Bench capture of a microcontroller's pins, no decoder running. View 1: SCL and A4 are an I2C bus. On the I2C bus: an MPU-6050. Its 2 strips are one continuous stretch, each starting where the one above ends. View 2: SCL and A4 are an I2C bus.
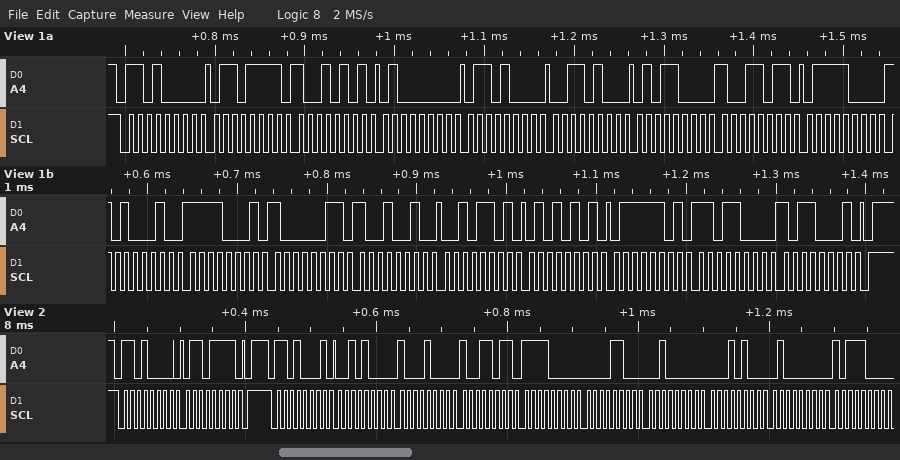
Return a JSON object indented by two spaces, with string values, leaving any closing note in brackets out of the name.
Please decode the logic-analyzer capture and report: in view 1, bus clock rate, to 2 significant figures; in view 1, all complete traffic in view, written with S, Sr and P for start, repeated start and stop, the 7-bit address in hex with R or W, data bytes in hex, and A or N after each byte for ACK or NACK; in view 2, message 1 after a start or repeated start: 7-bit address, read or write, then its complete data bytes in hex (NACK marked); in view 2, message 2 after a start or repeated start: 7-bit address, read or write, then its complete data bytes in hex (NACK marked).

{
  "in view 1, bus clock rate, to 2 significant figures": "100 kHz",
  "in view 1, all complete traffic in view, written with S, Sr and P for start, repeated start and stop, the 7-bit address in hex with R or W, data bytes in hex, and A or N after each byte for ACK or NACK": "S 68W A 6F A 95 A 40 A 68 A 34 A 58 A 9B A 78 A A2 A F1 A 83 A 92 A 2D A 55 A 7D A D8 A B1 A P",
  "in view 2, message 1 after a start or repeated start: 7-bit address, read or write, then its complete data bytes in hex": "0x68 write: 6F",
  "in view 2, message 2 after a start or repeated start: 7-bit address, read or write, then its complete data bytes in hex": "0x68 read: 28 88 9B F0 0C 20 14 40 B8"
}
